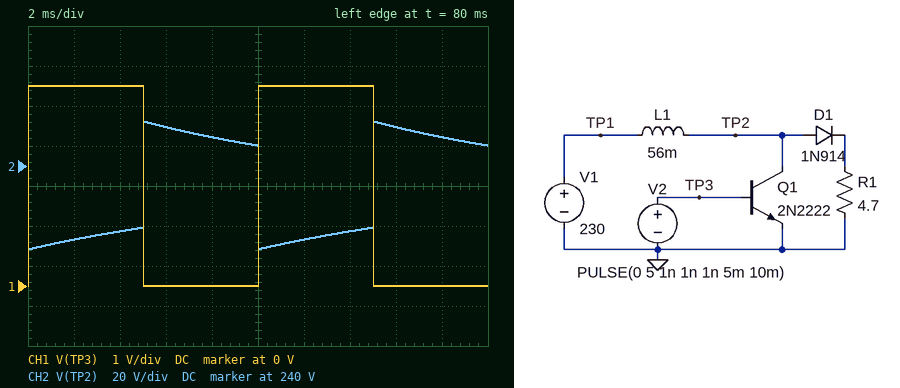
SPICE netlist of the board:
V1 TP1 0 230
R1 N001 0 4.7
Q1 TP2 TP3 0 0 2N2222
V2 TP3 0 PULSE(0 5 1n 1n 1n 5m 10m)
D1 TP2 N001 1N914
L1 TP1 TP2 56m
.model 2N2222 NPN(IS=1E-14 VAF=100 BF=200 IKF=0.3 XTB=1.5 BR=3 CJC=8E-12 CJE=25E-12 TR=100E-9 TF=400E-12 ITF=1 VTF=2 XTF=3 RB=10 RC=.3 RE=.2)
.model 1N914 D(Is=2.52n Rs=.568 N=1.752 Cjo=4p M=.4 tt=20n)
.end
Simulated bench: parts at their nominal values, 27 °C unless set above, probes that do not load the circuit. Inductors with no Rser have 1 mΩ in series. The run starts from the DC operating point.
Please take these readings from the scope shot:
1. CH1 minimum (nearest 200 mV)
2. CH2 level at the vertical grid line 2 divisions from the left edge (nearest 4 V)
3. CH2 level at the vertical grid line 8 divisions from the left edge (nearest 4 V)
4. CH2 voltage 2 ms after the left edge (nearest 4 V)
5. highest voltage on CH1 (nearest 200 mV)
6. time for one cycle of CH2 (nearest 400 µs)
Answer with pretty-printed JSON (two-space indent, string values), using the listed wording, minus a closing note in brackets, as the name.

{
  "CH1 minimum": "0 V",
  "CH2 level at the vertical grid line 2 divisions from the left edge": "208 V",
  "CH2 level at the vertical grid line 8 divisions from the left edge": "260 V",
  "CH2 voltage 2 ms after the left edge": "204 V",
  "highest voltage on CH1": "5.0 V",
  "time for one cycle of CH2": "10.0 ms"
}
